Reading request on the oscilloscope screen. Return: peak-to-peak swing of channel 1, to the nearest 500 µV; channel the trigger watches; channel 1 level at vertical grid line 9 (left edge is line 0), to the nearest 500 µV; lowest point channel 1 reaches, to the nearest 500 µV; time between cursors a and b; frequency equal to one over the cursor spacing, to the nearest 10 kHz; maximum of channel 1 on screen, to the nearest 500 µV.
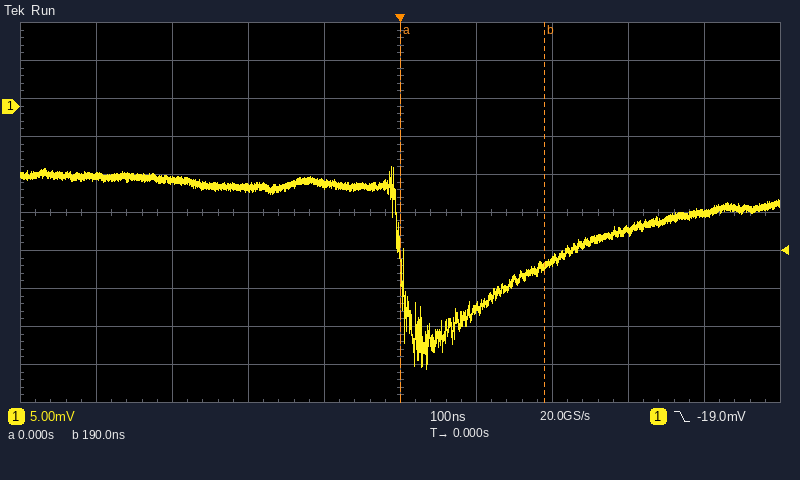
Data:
26.5 mV
channel 1
-14.0 mV
-34.5 mV
190 ns
5.26 MHz
-8.0 mV
